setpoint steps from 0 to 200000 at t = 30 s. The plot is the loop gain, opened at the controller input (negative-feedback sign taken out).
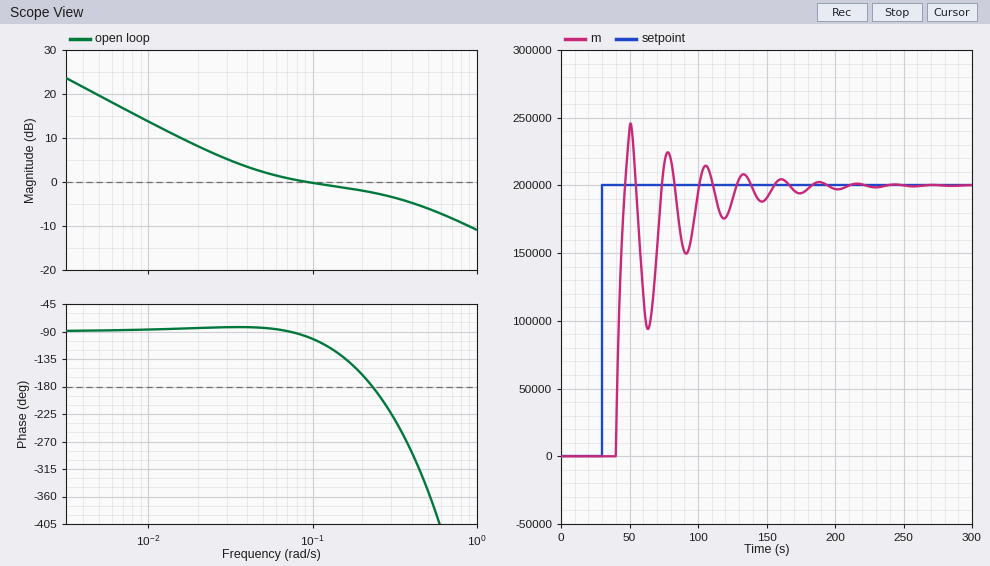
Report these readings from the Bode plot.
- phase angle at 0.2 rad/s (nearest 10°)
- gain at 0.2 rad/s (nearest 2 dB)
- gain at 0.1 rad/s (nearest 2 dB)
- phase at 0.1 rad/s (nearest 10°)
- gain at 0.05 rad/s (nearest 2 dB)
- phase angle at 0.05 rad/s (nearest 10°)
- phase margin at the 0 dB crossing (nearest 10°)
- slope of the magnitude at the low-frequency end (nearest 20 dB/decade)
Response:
-160°
-2 dB
0 dB
-100°
2 dB
-80°
80°
-20 dB/decade
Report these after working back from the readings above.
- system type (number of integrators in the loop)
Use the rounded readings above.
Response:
1
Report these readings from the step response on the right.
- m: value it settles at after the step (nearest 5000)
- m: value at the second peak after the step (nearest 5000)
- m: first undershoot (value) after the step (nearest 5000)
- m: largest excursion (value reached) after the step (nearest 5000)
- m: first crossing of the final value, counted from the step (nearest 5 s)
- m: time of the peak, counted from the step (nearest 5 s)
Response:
200000
225000
95000
245000
15 s
20 s
